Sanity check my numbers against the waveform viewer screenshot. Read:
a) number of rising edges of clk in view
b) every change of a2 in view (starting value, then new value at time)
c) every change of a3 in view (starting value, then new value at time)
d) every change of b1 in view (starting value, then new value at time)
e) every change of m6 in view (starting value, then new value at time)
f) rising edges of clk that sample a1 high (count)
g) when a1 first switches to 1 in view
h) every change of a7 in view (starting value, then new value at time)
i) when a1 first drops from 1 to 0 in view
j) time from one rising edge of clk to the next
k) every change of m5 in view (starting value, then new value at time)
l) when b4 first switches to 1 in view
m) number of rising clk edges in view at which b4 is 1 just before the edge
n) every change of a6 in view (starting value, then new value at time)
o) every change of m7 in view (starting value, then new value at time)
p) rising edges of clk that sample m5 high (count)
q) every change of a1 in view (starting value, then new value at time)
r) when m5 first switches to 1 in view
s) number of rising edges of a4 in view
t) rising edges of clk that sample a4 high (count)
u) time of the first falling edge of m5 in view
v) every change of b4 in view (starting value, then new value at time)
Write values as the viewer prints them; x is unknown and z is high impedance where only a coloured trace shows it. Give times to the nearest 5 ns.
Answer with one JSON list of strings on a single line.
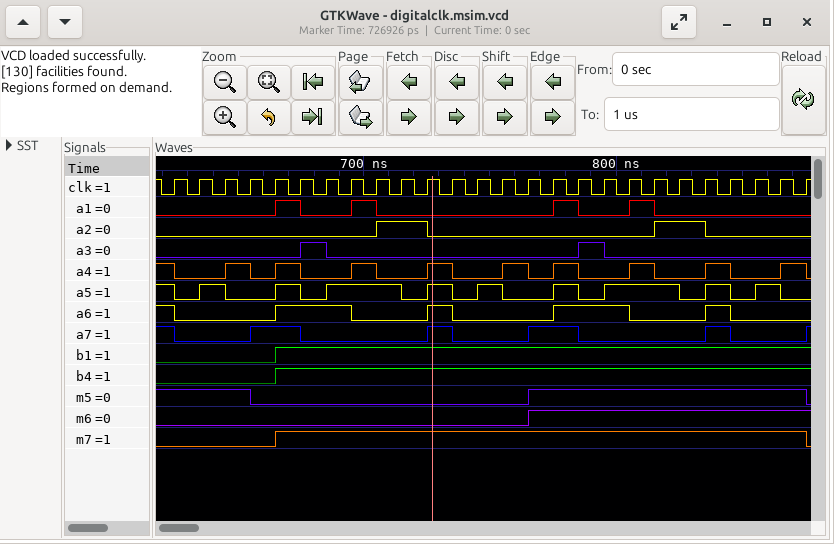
["26", "0, 1 at 705 ns, 0 at 725 ns, 1 at 815 ns, 0 at 835 ns", "0, 1 at 675 ns, 0 at 685 ns, 1 at 785 ns, 0 at 795 ns", "0, 1 at 665 ns", "0, 1 at 765 ns", "4", "665 ns", "1, 0 at 625 ns, 1 at 655 ns, 0 at 675 ns, 1 at 725 ns, 0 at 735 ns, 1 at 765 ns, 0 at 785 ns, 1 at 835 ns, 0 at 845 ns, 1 at 875 ns", "675 ns", "10 ns", "1, 0 at 655 ns, 1 at 765 ns, 0 at 875 ns", "665 ns", "21", "1, 0 at 625 ns, 1 at 665 ns, 0 at 695 ns, 1 at 725 ns, 0 at 735 ns, 1 at 775 ns, 0 at 805 ns, 1 at 835 ns, 0 at 845 ns", "0, 1 at 665 ns, 0 at 875 ns", "15", "0, 1 at 665 ns, 0 at 675 ns, 1 at 695 ns, 0 at 705 ns, 1 at 775 ns, 0 at 785 ns, 1 at 805 ns, 0 at 815 ns", "765 ns", "9", "10", "655 ns", "0, 1 at 665 ns"]
